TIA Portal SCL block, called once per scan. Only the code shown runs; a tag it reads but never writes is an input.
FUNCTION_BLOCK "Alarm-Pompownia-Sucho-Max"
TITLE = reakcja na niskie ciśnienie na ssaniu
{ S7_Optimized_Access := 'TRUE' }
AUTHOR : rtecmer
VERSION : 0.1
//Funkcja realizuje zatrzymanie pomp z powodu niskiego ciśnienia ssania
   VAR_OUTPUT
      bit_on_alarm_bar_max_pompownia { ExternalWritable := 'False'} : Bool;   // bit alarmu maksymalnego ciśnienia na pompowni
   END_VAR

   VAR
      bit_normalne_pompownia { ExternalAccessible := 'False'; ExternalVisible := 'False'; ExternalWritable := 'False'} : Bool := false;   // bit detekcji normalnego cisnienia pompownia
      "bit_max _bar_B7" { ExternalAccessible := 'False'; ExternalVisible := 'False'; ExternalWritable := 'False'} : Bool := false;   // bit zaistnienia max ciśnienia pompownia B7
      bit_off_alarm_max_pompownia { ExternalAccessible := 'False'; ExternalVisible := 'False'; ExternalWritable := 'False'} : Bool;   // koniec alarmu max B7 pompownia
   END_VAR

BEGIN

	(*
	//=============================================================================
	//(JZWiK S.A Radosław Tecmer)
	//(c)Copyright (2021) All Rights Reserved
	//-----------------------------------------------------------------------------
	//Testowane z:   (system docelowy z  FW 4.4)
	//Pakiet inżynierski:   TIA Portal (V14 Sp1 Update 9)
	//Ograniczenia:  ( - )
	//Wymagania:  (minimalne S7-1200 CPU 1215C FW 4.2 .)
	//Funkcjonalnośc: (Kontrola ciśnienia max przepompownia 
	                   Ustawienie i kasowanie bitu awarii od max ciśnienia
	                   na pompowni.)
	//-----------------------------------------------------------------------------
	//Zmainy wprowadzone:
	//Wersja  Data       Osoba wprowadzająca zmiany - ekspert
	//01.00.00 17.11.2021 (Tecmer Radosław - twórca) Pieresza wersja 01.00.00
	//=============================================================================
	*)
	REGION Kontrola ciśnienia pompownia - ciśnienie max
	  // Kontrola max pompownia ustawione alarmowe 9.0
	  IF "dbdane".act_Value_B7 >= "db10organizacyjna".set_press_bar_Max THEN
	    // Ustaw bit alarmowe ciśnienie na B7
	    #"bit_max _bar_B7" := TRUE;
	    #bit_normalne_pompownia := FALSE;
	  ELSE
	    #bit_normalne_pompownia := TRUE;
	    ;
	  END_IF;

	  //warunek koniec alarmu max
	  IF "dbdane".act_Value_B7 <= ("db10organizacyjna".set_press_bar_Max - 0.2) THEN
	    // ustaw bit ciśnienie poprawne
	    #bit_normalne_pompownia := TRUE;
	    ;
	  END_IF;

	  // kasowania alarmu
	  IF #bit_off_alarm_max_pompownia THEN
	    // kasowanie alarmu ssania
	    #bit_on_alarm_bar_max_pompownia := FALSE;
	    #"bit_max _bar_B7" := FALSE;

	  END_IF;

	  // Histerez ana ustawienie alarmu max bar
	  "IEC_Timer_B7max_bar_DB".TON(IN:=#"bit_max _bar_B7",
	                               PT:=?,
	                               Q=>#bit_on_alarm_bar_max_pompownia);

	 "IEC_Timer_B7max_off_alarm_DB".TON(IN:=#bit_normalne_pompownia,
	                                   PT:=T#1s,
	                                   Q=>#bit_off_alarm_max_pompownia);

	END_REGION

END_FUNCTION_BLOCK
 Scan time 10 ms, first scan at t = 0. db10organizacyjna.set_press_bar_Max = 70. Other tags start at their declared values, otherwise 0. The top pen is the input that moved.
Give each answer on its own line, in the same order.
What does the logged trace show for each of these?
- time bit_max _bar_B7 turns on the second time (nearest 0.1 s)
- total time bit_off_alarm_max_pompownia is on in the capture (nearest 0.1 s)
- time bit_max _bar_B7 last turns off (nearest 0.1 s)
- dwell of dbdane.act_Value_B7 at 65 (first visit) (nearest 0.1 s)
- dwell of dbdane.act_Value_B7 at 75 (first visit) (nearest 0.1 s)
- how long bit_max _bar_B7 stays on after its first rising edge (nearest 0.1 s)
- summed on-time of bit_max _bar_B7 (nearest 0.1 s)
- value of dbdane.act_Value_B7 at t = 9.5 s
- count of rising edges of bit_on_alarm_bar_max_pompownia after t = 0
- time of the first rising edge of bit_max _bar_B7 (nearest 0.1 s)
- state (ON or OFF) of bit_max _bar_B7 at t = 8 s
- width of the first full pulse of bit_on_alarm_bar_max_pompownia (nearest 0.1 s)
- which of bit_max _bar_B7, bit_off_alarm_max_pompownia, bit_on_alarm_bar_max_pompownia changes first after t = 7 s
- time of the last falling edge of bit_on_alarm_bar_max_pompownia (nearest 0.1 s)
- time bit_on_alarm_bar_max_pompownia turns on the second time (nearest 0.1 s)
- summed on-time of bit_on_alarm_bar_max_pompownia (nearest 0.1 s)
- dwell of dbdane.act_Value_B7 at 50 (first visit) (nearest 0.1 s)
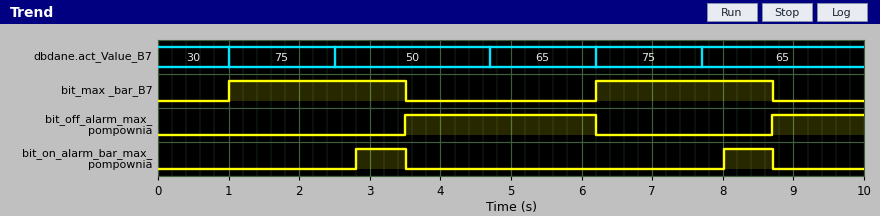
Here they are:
6.2 s
4.0 s
8.7 s
1.5 s
1.5 s
2.5 s
5.0 s
65
2
1.0 s
ON
0.7 s
bit_on_alarm_bar_max_pompownia
8.7 s
8.0 s
1.4 s
2.2 s
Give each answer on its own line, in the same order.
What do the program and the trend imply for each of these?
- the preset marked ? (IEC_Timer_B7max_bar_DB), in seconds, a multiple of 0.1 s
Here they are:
1.8 s
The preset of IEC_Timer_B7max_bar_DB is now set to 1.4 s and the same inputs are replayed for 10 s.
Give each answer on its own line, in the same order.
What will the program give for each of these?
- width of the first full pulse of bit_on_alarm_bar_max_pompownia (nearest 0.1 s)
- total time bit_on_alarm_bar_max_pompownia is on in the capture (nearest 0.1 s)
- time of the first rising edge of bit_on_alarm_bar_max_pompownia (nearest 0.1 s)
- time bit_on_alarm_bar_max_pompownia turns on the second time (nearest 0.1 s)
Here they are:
1.1 s
2.2 s
2.4 s
7.6 s
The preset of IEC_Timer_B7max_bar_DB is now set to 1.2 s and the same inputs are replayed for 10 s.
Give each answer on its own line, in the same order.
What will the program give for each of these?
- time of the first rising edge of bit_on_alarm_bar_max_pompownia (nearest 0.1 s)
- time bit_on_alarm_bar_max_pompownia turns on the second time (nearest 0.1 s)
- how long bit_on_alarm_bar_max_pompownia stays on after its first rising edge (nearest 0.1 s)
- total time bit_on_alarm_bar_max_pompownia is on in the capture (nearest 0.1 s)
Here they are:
2.2 s
7.4 s
1.3 s
2.6 s
